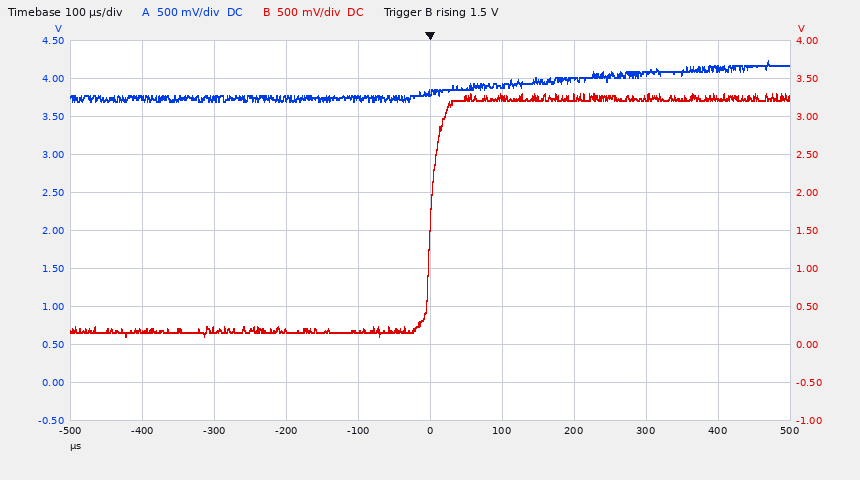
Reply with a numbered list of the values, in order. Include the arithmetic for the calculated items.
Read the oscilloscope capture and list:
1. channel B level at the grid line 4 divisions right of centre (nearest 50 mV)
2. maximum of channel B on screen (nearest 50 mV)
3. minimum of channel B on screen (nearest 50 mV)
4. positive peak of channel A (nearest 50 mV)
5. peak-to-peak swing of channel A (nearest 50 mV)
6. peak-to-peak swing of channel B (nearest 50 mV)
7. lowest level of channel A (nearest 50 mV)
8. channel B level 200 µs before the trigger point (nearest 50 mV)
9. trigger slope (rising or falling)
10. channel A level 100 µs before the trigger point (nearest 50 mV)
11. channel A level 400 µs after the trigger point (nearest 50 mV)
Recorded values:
1. 3.25 V
2. 3.30 V
3. 100 mV
4. 4.25 V
5. 4.25 V − (3.70 V) = 550 mV
6. 3.30 V − (100 mV) = 3.20 V
7. 3.70 V
8. 200 mV
9. rising
10. 3.75 V
11. 4.15 V
